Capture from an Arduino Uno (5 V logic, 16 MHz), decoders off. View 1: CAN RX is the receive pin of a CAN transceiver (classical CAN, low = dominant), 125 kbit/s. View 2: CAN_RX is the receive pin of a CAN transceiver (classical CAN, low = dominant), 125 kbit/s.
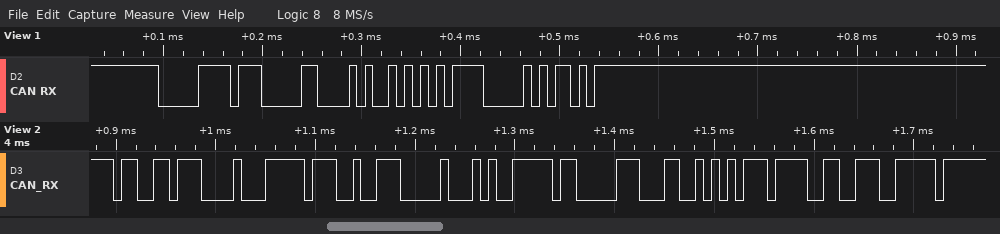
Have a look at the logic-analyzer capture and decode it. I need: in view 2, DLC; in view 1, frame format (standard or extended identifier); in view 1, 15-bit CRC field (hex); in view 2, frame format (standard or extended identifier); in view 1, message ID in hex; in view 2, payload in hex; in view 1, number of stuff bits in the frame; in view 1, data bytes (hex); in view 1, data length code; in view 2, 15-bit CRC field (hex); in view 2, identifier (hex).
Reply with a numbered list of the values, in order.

1. 8
2. standard
3. 0x7816
4. standard
5. 0x077
6. FF 27 00 A7 F0 63 2A EF
7. 3
8. 14 AA
9. 2
10. 0x19CF
11. 0x66E
